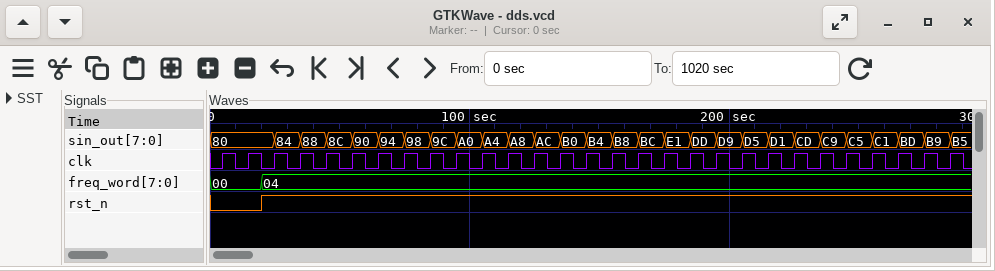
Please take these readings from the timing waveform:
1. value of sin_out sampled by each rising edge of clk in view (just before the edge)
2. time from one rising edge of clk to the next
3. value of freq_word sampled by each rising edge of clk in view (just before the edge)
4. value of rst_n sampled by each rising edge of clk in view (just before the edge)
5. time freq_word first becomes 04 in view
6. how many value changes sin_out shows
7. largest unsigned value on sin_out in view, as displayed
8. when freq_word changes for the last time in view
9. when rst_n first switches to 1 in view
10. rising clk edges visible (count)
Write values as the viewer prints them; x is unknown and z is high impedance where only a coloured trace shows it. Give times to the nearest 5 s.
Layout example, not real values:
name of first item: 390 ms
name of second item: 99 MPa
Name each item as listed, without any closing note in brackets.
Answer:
value of sin_out sampled by each rising edge of clk in view: 80, 80, 80, 84, 88, 8C, 90, 94, 98, 9C, A0, A4, A8, AC, B0, B4, B8, BC, E1, DD, D9, D5, D1, CD, C9, C5, C1, BD, B9
time from one rising edge of clk to the next: 10 s
value of freq_word sampled by each rising edge of clk in view: 00, 00, 04, 04, 04, 04, 04, 04, 04, 04, 04, 04, 04, 04, 04, 04, 04, 04, 04, 04, 04, 04, 04, 04, 04, 04, 04, 04, 04
value of rst_n sampled by each rising edge of clk in view: 0 0 1 1 1 1 1 1 1 1 1 1 1 1 1 1 1 1 1 1 1 1 1 1 1 1 1 1 1
time freq_word first becomes 04 in view: 20 s
how many value changes sin_out shows: 27
largest unsigned value on sin_out in view, as displayed: E1
when freq_word changes for the last time in view: 20 s
when rst_n first switches to 1 in view: 20 s
rising clk edges visible: 29
